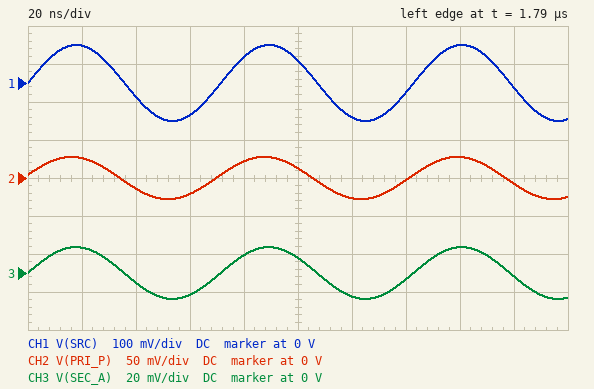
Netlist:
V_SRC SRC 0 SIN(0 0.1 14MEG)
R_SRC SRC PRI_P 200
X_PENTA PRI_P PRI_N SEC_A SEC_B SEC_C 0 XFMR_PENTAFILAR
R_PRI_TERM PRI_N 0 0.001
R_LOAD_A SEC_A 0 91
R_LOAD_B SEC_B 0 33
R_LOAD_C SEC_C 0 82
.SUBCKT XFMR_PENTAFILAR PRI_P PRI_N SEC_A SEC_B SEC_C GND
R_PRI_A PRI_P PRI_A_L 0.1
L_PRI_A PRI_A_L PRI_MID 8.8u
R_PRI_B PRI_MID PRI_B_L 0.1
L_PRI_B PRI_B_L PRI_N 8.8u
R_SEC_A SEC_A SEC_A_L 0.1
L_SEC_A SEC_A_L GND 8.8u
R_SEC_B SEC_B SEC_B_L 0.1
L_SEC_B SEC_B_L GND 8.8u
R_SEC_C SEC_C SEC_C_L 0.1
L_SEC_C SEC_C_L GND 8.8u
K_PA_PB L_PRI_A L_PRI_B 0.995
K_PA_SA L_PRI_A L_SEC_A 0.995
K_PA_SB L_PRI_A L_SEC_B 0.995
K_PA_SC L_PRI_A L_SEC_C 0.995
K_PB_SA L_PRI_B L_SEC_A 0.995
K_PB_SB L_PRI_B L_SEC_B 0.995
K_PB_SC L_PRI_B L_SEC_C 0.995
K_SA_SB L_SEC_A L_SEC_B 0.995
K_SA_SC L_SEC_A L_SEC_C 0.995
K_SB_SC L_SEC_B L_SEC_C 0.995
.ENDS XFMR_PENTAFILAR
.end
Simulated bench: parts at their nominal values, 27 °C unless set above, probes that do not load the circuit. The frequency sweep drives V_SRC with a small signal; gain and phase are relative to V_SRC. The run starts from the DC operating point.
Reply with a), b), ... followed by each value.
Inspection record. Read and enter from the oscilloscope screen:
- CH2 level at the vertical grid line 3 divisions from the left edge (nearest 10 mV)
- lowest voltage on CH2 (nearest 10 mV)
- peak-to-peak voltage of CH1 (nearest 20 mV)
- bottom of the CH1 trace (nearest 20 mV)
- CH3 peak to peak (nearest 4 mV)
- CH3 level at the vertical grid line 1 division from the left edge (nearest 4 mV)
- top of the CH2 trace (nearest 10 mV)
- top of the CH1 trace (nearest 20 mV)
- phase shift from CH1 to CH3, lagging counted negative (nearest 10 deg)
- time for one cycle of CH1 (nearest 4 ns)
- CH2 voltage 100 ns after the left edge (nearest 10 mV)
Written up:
a) -20 mV
b) -30 mV
c) 200 mV
d) -100 mV
e) 28 mV
f) 12 mV
g) 30 mV
h) 100 mV
i) 0 deg
j) 72 ns
k) 10 mV
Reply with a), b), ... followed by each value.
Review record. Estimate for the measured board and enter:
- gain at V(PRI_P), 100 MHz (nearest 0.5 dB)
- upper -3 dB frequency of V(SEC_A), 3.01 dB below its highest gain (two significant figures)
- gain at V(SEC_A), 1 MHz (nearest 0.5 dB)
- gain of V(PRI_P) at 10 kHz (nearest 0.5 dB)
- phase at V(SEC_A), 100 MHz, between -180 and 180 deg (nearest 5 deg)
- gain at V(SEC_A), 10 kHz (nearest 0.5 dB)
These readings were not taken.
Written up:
a) -7.5 dB
b) 500 MHz
c) -17.5 dB
d) -39.0 dB
e) -5 deg
f) -45.0 dB
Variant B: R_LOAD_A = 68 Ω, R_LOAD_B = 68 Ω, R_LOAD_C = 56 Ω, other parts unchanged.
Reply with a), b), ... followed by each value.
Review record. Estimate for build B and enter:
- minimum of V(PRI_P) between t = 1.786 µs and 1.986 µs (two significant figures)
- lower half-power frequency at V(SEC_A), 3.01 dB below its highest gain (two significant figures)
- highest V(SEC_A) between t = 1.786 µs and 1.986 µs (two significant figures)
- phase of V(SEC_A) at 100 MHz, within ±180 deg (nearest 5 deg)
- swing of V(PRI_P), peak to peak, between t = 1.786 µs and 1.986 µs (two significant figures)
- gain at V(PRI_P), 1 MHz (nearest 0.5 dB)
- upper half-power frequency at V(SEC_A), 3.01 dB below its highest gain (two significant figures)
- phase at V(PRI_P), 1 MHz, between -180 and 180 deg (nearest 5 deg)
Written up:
a) -30 mV
b) 270 kHz
c) 15 mV
d) -15 deg
e) 60 mV
f) -11.0 dB
g) 340 MHz
h) 15 deg
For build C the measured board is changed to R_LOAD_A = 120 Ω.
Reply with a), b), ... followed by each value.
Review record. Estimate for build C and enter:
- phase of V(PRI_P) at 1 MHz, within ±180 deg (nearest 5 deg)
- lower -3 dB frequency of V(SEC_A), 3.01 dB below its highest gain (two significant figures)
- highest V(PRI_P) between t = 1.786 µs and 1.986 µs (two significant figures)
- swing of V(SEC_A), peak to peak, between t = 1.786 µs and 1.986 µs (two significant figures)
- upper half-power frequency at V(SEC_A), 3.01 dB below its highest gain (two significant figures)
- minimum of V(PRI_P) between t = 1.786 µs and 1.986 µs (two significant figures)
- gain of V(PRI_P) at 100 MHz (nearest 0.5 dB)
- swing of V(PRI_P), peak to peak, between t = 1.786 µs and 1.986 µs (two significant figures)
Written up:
a) 15 deg
b) 350 kHz
c) 29 mV
d) 28 mV
e) 610 MHz
f) -29 mV
g) -7.0 dB
h) 58 mV
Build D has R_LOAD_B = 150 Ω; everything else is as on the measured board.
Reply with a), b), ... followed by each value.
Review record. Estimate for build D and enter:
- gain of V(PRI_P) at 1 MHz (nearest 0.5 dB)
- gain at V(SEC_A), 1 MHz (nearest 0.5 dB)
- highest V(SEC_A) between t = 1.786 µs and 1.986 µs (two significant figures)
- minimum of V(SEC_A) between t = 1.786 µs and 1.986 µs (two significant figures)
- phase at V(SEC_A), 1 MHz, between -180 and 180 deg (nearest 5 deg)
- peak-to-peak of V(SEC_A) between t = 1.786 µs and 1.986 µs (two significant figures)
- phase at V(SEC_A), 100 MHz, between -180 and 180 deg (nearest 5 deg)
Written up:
a) -8.5 dB
b) -14.5 dB
c) 20 mV
d) -20 mV
e) 20 deg
f) 40 mV
g) -15 deg
